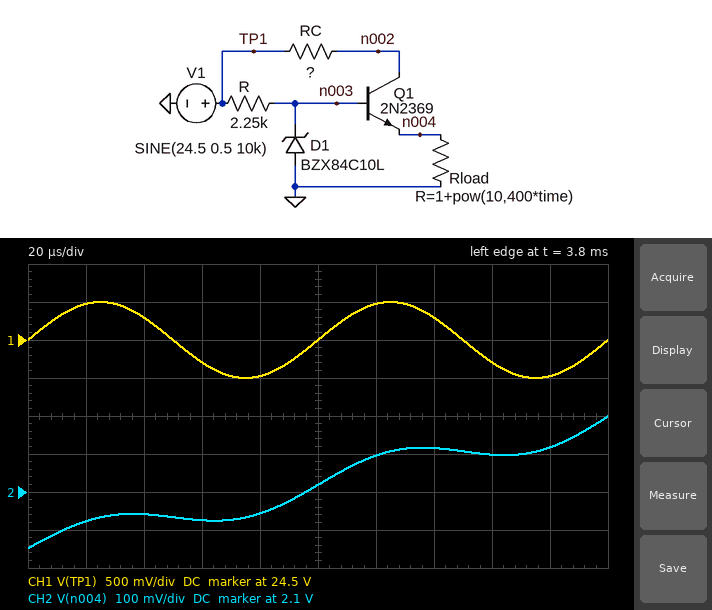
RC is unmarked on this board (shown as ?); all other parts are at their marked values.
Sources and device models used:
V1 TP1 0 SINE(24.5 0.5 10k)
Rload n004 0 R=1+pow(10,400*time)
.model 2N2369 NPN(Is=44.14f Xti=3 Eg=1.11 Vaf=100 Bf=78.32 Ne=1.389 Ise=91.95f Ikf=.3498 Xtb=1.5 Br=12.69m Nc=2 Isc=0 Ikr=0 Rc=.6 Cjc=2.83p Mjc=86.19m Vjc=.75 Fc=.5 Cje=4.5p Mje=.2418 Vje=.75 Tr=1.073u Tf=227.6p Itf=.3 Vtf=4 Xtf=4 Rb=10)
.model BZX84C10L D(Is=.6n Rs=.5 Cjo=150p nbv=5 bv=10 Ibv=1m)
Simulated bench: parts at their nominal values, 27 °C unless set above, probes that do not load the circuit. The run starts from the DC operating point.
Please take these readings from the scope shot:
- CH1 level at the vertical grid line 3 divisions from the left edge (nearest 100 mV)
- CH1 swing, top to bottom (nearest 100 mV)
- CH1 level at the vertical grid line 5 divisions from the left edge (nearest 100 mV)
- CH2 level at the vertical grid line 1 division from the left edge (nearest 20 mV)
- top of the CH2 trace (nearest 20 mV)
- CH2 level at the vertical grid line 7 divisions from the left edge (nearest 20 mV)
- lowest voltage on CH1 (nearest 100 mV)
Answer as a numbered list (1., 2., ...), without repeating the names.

1. 24.2 V
2. 1.0 V
3. 24.5 V
4. 2.02 V
5. 2.30 V
6. 2.22 V
7. 24.0 V
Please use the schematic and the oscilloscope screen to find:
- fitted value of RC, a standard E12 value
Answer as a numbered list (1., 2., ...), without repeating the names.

1. 470 Ω
